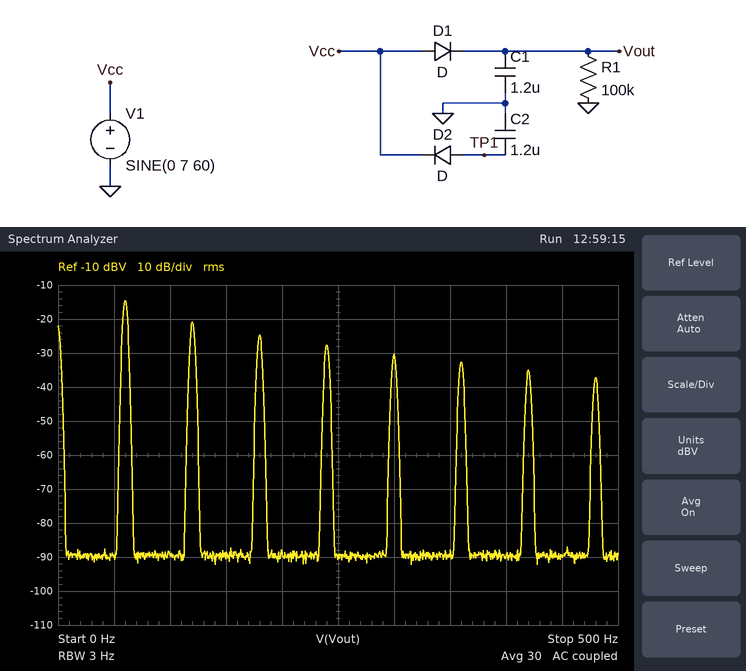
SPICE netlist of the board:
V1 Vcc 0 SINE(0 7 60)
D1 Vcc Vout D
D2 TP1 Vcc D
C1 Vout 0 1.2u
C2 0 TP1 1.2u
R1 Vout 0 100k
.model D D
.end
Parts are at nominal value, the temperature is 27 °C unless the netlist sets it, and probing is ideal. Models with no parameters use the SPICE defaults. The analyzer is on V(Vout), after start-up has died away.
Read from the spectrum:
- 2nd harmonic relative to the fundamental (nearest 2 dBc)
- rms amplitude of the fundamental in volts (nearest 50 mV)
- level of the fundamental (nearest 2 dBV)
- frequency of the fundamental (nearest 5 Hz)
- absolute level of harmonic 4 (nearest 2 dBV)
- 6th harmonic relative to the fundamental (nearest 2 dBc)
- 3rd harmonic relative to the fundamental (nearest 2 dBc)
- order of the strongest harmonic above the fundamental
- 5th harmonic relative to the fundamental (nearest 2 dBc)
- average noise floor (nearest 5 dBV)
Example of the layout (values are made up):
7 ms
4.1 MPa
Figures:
-6 dBc
200 mV
-14 dBV
60 Hz
-28 dBV
-18 dBc
-10 dBc
2
-16 dBc
-90 dBV
